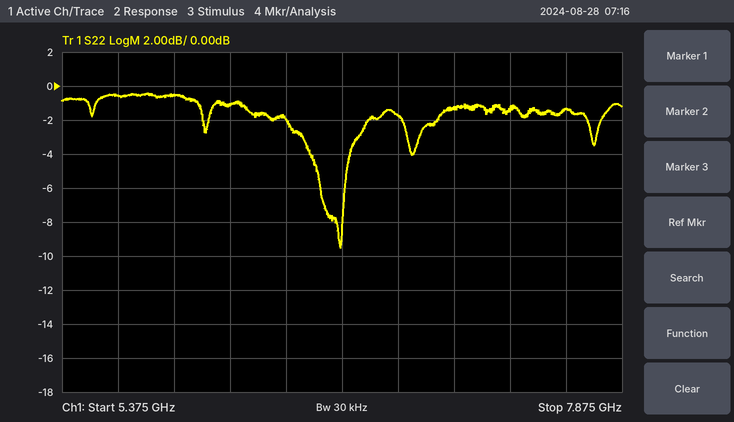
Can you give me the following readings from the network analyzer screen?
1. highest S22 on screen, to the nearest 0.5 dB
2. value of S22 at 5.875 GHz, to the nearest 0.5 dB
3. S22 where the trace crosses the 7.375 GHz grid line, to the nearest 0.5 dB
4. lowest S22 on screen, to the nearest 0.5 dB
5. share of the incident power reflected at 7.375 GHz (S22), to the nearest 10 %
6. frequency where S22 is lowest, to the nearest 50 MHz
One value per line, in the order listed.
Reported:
-0.5 dB
-0.5 dB
-1.5 dB
-9.5 dB
70 %
6.60 GHz
